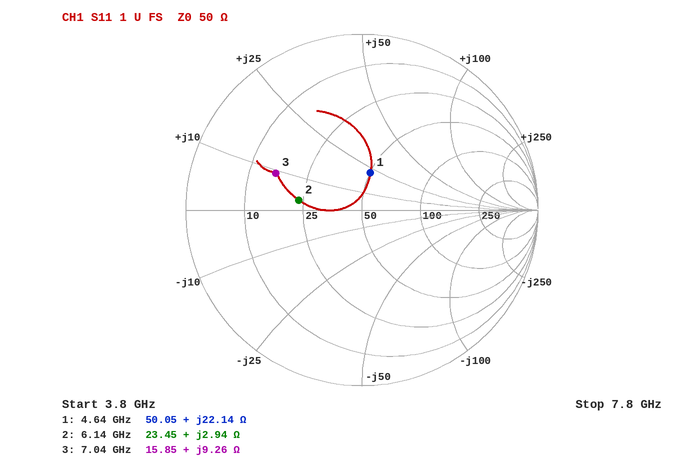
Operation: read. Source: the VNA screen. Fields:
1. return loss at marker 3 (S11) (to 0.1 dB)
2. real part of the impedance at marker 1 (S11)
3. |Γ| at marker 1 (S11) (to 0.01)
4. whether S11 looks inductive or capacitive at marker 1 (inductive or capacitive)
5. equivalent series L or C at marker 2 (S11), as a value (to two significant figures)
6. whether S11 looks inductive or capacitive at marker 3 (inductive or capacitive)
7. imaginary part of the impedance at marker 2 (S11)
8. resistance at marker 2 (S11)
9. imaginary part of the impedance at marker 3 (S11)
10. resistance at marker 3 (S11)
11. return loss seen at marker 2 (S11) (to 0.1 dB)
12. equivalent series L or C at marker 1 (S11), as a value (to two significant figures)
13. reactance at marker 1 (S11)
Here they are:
5.5 dB
50.05 Ω
0.22
inductive
76 pH
inductive
+2.94 Ω
23.45 Ω
+9.26 Ω
15.85 Ω
8.8 dB
760 pH
+22.14 Ω
